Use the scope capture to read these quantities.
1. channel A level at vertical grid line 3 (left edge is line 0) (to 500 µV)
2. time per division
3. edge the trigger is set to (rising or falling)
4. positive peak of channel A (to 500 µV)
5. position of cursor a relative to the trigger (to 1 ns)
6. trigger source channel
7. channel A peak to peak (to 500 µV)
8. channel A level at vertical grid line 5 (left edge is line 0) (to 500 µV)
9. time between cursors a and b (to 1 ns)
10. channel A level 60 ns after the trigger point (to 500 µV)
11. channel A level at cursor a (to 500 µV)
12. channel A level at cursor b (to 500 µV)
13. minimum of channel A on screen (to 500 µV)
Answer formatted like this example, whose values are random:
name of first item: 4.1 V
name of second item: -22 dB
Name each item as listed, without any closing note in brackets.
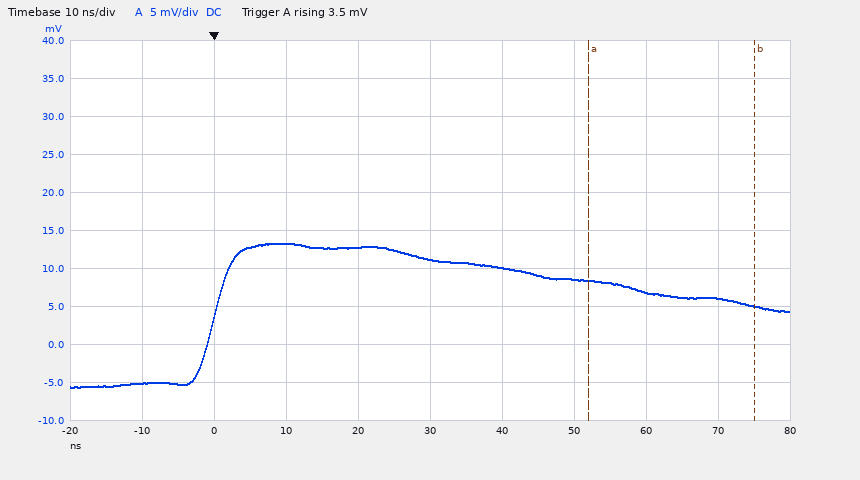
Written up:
channel A level at vertical grid line 3 (left edge is line 0): 13.5 mV
time per division: 10 ns
edge the trigger is set to: rising
positive peak of channel A: 13.5 mV
position of cursor a relative to the trigger: +52 ns
trigger source channel: channel A
channel A peak to peak: 19.0 mV
channel A level at vertical grid line 5 (left edge is line 0): 11.0 mV
time between cursors a and b: 23 ns
channel A level 60 ns after the trigger point: 7.0 mV
channel A level at cursor a: 8.5 mV
channel A level at cursor b: 5.0 mV
minimum of channel A on screen: -5.5 mV
